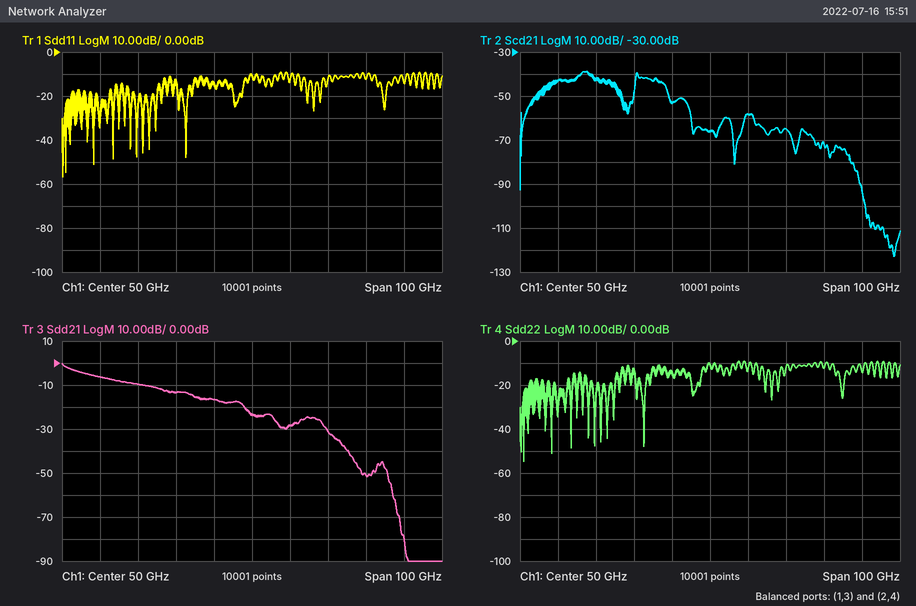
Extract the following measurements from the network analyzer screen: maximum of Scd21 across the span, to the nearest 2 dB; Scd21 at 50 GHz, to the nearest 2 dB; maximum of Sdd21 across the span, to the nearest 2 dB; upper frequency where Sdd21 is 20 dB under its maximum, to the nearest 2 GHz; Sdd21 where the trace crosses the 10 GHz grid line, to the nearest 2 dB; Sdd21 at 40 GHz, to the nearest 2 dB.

-38 dB
-66 dB
0 dB
48 GHz
-6 dB
-16 dB
